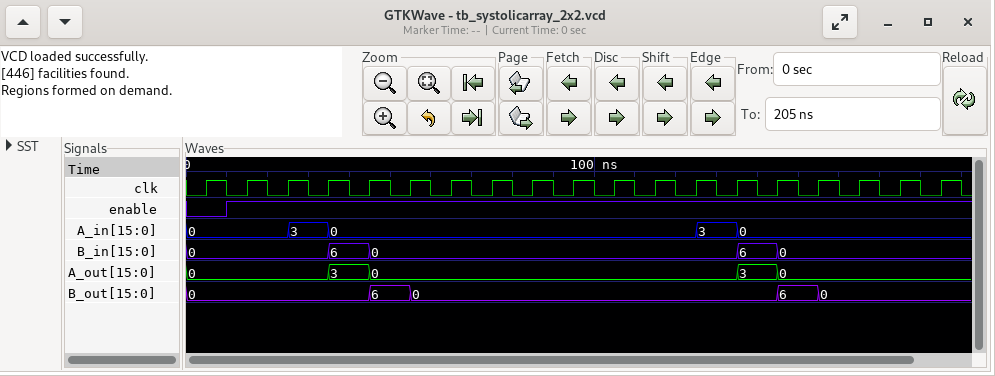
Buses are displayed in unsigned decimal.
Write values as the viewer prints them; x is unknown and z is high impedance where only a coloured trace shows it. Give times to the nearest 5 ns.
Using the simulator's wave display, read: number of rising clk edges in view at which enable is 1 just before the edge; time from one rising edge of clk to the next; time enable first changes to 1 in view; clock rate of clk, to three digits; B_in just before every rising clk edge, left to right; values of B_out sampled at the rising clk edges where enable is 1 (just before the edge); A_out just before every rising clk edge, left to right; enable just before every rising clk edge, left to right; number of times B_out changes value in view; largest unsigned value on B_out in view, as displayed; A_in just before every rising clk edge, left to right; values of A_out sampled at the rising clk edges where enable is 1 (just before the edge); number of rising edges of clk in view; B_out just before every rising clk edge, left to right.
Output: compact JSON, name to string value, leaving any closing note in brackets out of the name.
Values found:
{"number of rising clk edges in view at which enable is 1 just before the edge": "18", "time from one rising edge of clk to the next": "10 ns", "time enable first changes to 1 in view": "10 ns", "clock rate of clk, to three digits": "100 MHz", "B_in just before every rising clk edge, left to right": "0, 0, 0, 0, 6, 0, 0, 0, 0, 0, 0, 0, 0, 0, 6, 0, 0, 0, 0", "values of B_out sampled at the rising clk edges where enable is 1": "0, 0, 0, 0, 6, 0, 0, 0, 0, 0, 0, 0, 0, 0, 6, 0, 0, 0", "A_out just before every rising clk edge, left to right": "0, 0, 0, 0, 3, 0, 0, 0, 0, 0, 0, 0, 0, 0, 3, 0, 0, 0, 0", "enable just before every rising clk edge, left to right": "0 1 1 1 1 1 1 1 1 1 1 1 1 1 1 1 1 1 1", "number of times B_out changes value in view": "4", "largest unsigned value on B_out in view, as displayed": "6", "A_in just before every rising clk edge, left to right": "0, 0, 0, 3, 0, 0, 0, 0, 0, 0, 0, 0, 0, 3, 0, 0, 0, 0, 0", "values of A_out sampled at the rising clk edges where enable is 1": "0, 0, 0, 3, 0, 0, 0, 0, 0, 0, 0, 0, 0, 3, 0, 0, 0, 0", "number of rising edges of clk in view": "19", "B_out just before every rising clk edge, left to right": "0, 0, 0, 0, 0, 6, 0, 0, 0, 0, 0, 0, 0, 0, 0, 6, 0, 0, 0"}
